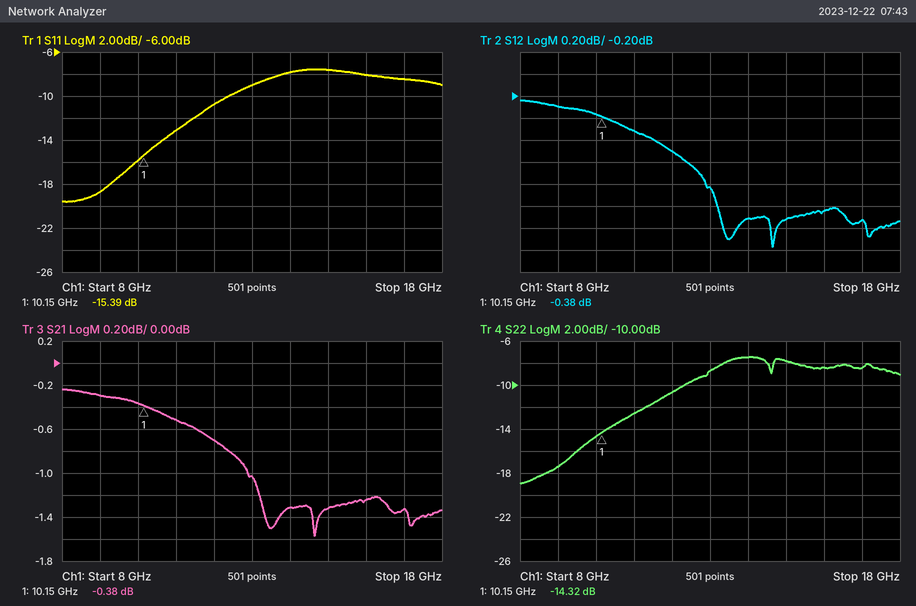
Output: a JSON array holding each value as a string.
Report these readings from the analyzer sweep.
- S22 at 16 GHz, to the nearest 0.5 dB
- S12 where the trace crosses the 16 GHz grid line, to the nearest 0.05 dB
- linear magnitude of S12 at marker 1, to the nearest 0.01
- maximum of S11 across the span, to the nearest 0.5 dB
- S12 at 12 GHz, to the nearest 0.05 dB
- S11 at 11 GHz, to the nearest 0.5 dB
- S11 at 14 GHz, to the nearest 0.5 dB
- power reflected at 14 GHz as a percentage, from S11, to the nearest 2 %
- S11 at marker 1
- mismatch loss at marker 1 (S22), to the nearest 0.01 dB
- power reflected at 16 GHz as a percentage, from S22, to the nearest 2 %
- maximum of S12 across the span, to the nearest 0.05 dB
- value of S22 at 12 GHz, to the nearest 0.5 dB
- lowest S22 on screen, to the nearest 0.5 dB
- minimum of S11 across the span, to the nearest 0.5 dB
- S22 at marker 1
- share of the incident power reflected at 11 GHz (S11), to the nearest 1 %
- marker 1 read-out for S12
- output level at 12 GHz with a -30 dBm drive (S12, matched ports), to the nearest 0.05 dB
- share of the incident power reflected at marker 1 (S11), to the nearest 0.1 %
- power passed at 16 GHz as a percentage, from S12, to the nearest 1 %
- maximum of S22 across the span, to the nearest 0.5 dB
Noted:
["-8.5 dB", "-1.25 dB", "0.96", "-7.5 dB", "-0.70 dB", "-13.0 dB", "-8.0 dB", "16 %", "-15.39 dB", "0.16 dB", "14 %", "-0.25 dB", "-10.5 dB", "-19.0 dB", "-19.5 dB", "-14.32 dB", "5 %", "-0.38 dB", "-30.70 dBm", "2.9 %", "75 %", "-7.5 dB"]
